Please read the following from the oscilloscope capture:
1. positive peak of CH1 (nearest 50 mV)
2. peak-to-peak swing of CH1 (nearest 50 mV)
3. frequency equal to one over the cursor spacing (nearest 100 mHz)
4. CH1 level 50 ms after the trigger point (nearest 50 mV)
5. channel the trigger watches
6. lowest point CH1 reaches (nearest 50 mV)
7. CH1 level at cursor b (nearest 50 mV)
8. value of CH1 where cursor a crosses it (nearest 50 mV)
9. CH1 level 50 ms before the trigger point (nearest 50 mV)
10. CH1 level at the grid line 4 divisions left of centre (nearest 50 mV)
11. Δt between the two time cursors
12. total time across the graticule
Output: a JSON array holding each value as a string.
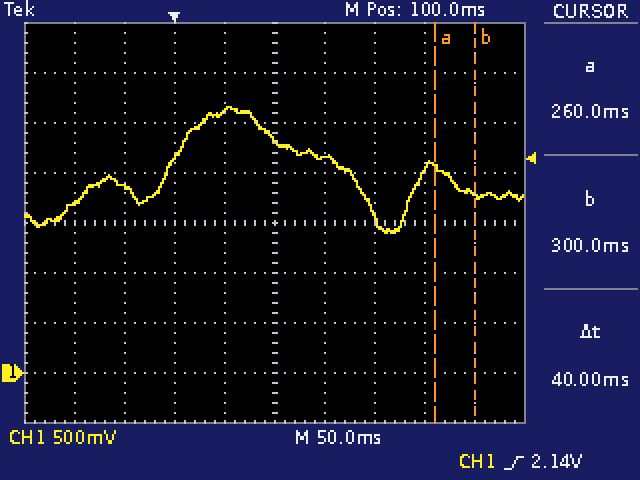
["2.65 V", "1.25 V", "25.0 Hz", "2.60 V", "CH1", "1.40 V", "1.80 V", "2.05 V", "1.85 V", "1.70 V", "40 ms", "500 ms"]
